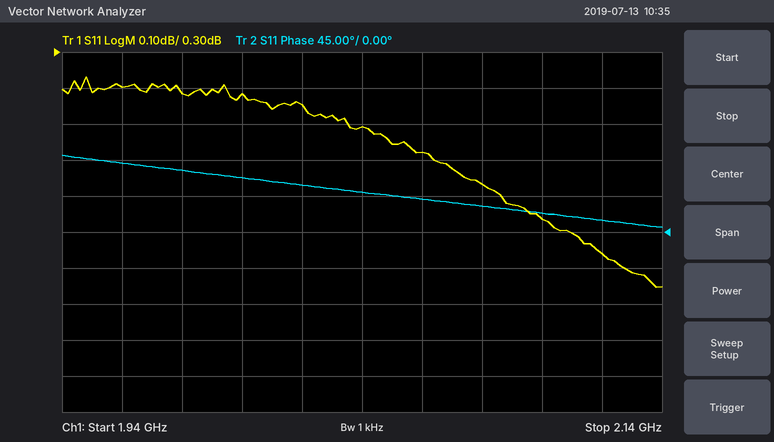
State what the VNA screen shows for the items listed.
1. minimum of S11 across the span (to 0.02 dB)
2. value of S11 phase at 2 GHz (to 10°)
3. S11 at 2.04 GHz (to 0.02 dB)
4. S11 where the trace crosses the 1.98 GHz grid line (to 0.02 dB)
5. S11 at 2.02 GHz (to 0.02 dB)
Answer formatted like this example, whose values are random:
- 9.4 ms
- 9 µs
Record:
- -0.36 dB
- 70°
- 0.10 dB
- 0.18 dB
- 0.16 dB
